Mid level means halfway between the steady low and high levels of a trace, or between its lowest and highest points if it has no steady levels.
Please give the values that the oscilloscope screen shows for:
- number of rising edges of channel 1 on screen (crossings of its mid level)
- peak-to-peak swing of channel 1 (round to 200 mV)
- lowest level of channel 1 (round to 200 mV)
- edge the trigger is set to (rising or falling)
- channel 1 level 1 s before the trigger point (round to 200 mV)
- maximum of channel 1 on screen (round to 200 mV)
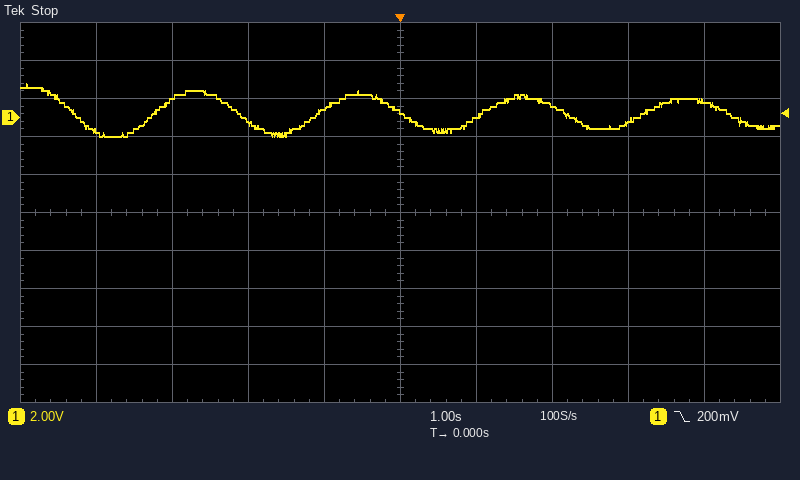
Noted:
4
2.8 V
-1.0 V
falling
400 mV
1.8 V
